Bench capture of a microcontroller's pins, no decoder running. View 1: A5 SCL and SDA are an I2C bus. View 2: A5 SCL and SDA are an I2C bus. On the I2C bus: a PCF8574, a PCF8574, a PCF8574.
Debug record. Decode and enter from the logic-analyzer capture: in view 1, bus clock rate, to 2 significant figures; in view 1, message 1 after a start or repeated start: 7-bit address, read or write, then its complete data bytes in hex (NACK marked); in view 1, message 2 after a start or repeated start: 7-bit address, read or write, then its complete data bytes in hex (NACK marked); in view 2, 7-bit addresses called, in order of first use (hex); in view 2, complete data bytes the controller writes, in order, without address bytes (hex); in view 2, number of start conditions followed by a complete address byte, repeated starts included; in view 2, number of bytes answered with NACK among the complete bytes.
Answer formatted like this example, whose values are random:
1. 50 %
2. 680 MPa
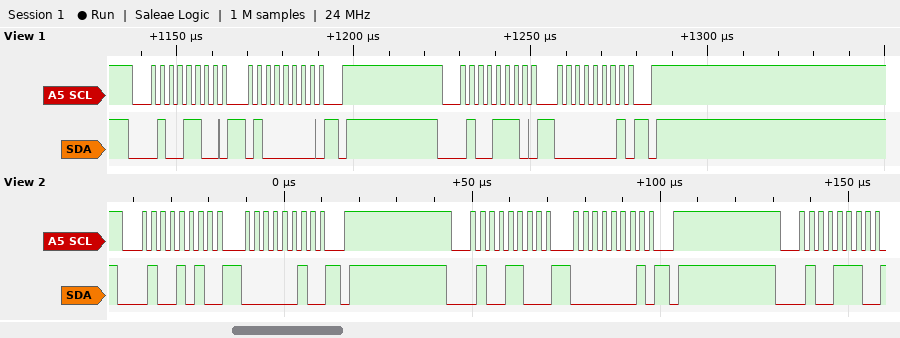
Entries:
1. 400 kHz
2. 0x26 write: 40
3. 0x27 write: 01
4. 0x25 0x26 0x27
5. 02 01
6. 3
7. 0
